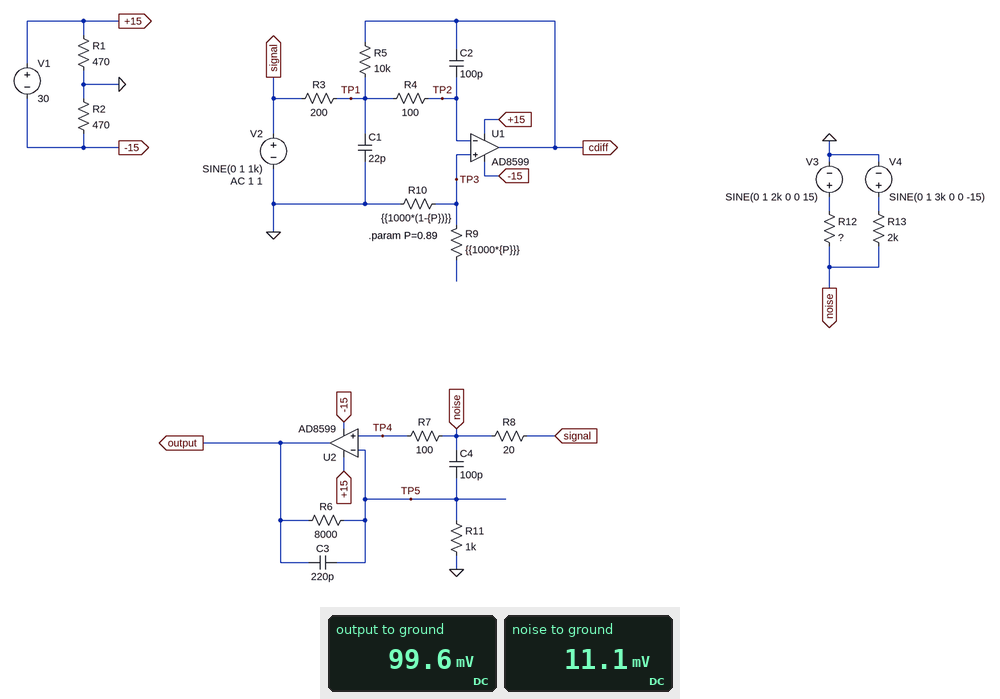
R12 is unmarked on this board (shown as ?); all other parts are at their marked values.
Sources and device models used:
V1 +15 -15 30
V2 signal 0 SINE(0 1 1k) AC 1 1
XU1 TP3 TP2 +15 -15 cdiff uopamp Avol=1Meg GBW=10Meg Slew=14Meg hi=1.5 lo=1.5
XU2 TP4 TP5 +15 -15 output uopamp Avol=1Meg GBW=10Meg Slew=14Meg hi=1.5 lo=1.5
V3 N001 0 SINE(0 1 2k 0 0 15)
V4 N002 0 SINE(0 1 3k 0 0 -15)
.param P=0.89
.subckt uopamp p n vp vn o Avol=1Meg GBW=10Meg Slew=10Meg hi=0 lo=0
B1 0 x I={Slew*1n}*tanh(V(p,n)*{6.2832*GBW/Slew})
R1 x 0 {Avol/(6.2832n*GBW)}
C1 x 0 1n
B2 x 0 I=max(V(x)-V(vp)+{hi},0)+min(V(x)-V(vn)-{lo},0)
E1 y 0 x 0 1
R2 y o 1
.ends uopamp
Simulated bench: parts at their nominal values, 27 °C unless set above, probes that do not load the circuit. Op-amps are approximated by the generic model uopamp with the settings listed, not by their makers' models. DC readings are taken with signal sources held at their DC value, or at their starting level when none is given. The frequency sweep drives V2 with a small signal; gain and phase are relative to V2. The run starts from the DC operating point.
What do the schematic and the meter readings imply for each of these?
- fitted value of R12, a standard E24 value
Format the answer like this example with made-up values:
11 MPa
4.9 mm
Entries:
360 Ω
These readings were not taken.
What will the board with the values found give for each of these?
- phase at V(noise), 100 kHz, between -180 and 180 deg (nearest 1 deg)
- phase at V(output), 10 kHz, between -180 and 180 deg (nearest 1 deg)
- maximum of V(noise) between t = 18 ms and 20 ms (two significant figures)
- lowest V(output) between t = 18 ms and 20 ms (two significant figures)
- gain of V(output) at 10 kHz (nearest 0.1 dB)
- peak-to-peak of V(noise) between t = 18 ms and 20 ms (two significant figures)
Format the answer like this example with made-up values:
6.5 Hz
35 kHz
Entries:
0 deg
-6 deg
920 mV
-8.5 V
18.5 dB
1.9 V
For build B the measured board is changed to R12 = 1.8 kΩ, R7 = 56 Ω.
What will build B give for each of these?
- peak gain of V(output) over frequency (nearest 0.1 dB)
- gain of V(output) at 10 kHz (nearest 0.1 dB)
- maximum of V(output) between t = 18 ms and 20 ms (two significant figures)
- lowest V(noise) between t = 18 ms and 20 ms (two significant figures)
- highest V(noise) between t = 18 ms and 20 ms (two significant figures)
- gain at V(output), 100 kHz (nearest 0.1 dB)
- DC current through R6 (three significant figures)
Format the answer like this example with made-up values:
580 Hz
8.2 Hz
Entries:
18.9 dB
18.8 dB
8.7 V
-970 mV
970 mV
15.2 dB
282 nA
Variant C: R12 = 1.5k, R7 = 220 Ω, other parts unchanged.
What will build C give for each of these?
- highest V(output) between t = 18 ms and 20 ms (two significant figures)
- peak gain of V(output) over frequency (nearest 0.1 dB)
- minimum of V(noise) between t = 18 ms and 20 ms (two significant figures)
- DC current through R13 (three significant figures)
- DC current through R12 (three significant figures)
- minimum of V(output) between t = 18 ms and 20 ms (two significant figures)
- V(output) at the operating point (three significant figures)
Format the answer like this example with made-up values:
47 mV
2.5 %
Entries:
8.7 V
18.9 dB
-970 mV
130 µA
172 µA
-8.7 V
7.59 mV
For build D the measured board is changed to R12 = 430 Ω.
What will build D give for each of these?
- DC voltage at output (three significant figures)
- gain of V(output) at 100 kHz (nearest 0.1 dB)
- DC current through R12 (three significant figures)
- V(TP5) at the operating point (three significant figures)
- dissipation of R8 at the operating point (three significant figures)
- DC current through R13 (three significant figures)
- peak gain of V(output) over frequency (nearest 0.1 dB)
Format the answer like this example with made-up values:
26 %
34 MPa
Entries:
80.5 mV
14.9 dB
581 µA
8.94 mV
4.00 µW
134 µA
18.6 dB
